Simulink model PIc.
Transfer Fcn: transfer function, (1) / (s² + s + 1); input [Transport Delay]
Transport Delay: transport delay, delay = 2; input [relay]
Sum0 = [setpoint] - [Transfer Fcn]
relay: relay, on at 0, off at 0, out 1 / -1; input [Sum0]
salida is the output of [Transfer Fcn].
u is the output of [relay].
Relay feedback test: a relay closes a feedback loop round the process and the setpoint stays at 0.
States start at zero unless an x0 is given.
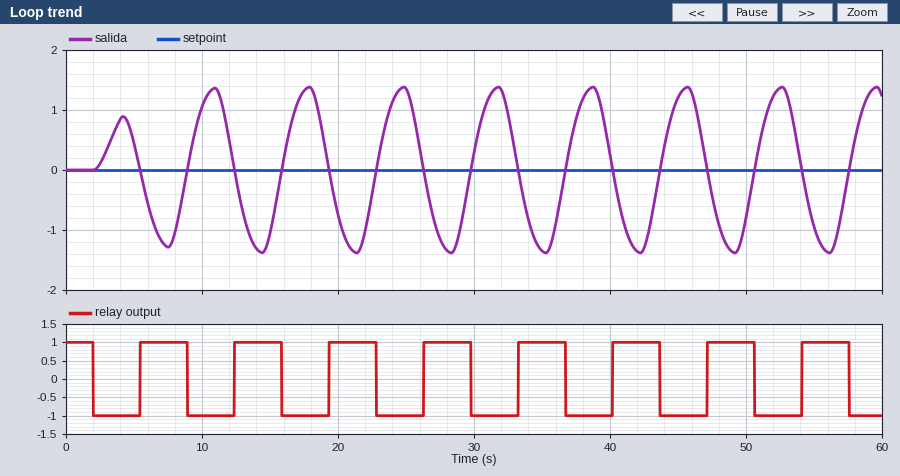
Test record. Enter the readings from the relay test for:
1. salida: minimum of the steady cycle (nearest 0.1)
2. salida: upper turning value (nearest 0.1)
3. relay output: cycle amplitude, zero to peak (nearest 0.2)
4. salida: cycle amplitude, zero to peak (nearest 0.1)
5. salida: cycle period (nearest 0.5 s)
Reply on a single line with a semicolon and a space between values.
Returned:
-1.4; 1.4; 1.0; 1.4; 7.0 s
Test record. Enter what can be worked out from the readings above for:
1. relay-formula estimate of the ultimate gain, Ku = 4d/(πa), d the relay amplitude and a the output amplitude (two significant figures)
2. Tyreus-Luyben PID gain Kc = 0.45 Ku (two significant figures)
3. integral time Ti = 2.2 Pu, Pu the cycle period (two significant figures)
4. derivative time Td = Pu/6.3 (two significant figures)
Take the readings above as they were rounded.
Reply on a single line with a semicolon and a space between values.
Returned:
0.91; 0.41; 15 s; 1.1 s
